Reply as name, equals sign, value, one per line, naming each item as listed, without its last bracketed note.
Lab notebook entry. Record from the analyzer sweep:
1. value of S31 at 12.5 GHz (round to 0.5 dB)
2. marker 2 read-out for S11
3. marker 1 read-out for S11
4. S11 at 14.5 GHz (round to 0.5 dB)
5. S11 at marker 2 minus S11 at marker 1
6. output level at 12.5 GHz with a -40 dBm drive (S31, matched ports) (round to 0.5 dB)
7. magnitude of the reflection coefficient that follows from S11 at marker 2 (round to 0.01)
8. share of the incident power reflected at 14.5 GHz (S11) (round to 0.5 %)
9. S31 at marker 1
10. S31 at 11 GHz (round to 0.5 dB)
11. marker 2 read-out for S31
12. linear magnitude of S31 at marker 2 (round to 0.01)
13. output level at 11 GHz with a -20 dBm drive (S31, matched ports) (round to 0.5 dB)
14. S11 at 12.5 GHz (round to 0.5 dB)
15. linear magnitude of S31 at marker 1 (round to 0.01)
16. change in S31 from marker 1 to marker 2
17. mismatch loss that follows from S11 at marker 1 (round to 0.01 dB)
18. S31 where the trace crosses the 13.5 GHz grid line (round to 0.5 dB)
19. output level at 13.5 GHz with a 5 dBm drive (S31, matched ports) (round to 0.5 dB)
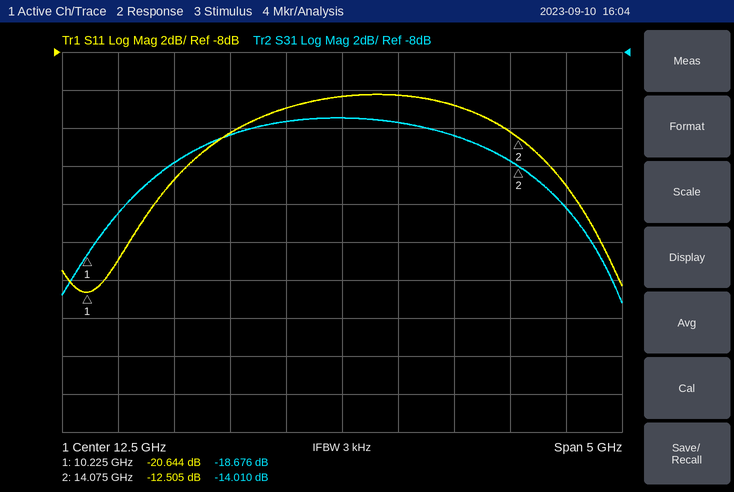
value of S31 at 12.5 GHz = -11.5 dB
marker 2 read-out for S11 = -12.505 dB
marker 1 read-out for S11 = -20.644 dB
S11 at 14.5 GHz = -15.0 dB
S11 at marker 2 minus S11 at marker 1 = 8.139 dB
output level at 12.5 GHz with a -40 dBm drive (S31, matched ports) = -51.5 dBm
magnitude of the reflection coefficient that follows from S11 at marker 2 = 0.24
share of the incident power reflected at 14.5 GHz (S11) = 3.0 %
S31 at marker 1 = -18.676 dB
S31 at 11 GHz = -14.0 dB
marker 2 read-out for S31 = -14.010 dB
linear magnitude of S31 at marker 2 = 0.20
output level at 11 GHz with a -20 dBm drive (S31, matched ports) = -34.0 dBm
S11 at 12.5 GHz = -10.5 dB
linear magnitude of S31 at marker 1 = 0.12
change in S31 from marker 1 to marker 2 = 4.666 dB
mismatch loss that follows from S11 at marker 1 = 0.04 dB
S31 where the trace crosses the 13.5 GHz grid line = -12.5 dB
output level at 13.5 GHz with a 5 dBm drive (S31, matched ports) = -7.5 dBm
